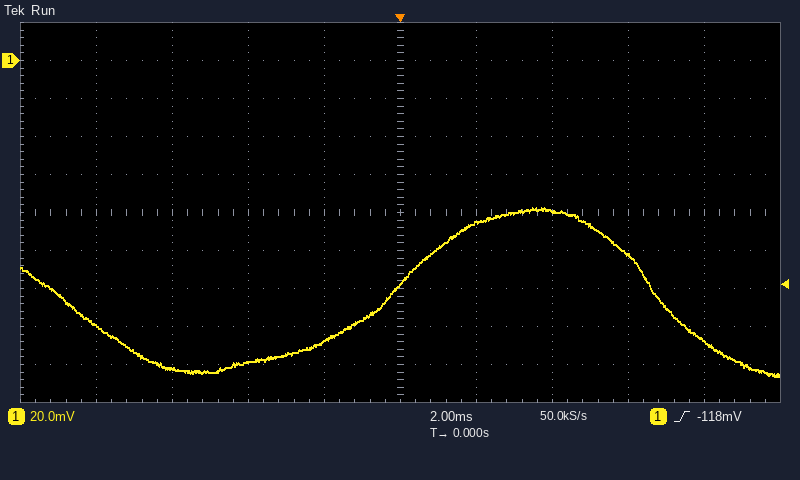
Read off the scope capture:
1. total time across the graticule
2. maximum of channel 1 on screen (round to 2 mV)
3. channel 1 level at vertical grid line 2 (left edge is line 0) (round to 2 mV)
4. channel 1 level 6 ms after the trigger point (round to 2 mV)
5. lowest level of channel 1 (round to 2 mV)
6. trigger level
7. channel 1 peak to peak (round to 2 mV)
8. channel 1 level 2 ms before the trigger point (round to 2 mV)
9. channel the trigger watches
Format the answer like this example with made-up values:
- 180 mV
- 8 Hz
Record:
- 20 ms
- -78 mV
- -162 mV
- -102 mV
- -166 mV
- -118 mV
- 88 mV
- -148 mV
- channel 1
